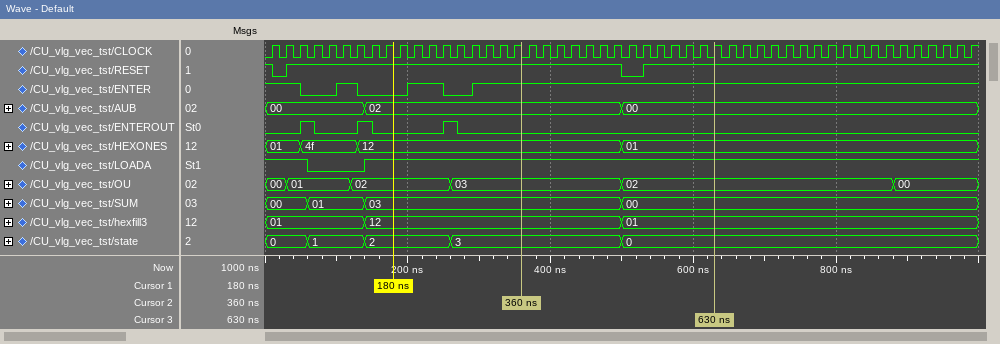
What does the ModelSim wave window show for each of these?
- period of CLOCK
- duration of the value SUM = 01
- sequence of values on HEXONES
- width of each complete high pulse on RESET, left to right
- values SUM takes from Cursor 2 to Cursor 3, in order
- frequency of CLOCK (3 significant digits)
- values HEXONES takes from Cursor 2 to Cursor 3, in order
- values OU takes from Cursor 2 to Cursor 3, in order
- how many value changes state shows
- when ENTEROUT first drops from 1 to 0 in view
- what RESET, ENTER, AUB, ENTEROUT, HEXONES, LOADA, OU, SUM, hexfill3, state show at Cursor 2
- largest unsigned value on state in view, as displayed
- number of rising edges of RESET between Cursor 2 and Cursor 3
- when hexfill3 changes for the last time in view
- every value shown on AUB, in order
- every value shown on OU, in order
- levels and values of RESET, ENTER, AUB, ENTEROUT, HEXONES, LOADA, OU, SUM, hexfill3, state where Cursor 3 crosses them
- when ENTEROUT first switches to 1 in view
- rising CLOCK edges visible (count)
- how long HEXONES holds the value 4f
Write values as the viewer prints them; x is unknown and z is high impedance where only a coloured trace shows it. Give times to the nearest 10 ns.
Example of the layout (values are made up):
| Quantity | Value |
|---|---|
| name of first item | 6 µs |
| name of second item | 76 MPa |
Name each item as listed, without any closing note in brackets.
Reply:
| Quantity | Value |
|---|---|
| period of CLOCK | 20 ns |
| duration of the value SUM = 01 | 80 ns |
| sequence of values on HEXONES | 01, 4f, 12, 01 |
| width of each complete high pulse on RESET, left to right | 470 ns |
| values SUM takes from Cursor 2 to Cursor 3, in order | 03, 00 |
| frequency of CLOCK | 50.0 MHz |
| values HEXONES takes from Cursor 2 to Cursor 3, in order | 12, 01 |
| values OU takes from Cursor 2 to Cursor 3, in order | 03, 02 |
| how many value changes state shows | 4 |
| when ENTEROUT first drops from 1 to 0 in view | 70 ns |
| what RESET, ENTER, AUB, ENTEROUT, HEXONES, LOADA, OU, SUM, hexfill3, state show at Cursor 2 | RESET=1, ENTER=1, AUB=02, ENTEROUT=0, HEXONES=12, LOADA=1, OU=03, SUM=03, hexfill3=12, state=3 |
| largest unsigned value on state in view, as displayed | 3 |
| number of rising edges of RESET between Cursor 2 and Cursor 3 | 1 |
| when hexfill3 changes for the last time in view | 500 ns |
| every value shown on AUB, in order | 00, 02, 00 |
| every value shown on OU, in order | 00, 01, 02, 03, 02, 00 |
| levels and values of RESET, ENTER, AUB, ENTEROUT, HEXONES, LOADA, OU, SUM, hexfill3, state where Cursor 3 crosses them | RESET=1, ENTER=1, AUB=00, ENTEROUT=0, HEXONES=01, LOADA=1, OU=02, SUM=00, hexfill3=01, state=0 |
| when ENTEROUT first switches to 1 in view | 50 ns |
| rising CLOCK edges visible | 50 |
| how long HEXONES holds the value 4f | 80 ns |
